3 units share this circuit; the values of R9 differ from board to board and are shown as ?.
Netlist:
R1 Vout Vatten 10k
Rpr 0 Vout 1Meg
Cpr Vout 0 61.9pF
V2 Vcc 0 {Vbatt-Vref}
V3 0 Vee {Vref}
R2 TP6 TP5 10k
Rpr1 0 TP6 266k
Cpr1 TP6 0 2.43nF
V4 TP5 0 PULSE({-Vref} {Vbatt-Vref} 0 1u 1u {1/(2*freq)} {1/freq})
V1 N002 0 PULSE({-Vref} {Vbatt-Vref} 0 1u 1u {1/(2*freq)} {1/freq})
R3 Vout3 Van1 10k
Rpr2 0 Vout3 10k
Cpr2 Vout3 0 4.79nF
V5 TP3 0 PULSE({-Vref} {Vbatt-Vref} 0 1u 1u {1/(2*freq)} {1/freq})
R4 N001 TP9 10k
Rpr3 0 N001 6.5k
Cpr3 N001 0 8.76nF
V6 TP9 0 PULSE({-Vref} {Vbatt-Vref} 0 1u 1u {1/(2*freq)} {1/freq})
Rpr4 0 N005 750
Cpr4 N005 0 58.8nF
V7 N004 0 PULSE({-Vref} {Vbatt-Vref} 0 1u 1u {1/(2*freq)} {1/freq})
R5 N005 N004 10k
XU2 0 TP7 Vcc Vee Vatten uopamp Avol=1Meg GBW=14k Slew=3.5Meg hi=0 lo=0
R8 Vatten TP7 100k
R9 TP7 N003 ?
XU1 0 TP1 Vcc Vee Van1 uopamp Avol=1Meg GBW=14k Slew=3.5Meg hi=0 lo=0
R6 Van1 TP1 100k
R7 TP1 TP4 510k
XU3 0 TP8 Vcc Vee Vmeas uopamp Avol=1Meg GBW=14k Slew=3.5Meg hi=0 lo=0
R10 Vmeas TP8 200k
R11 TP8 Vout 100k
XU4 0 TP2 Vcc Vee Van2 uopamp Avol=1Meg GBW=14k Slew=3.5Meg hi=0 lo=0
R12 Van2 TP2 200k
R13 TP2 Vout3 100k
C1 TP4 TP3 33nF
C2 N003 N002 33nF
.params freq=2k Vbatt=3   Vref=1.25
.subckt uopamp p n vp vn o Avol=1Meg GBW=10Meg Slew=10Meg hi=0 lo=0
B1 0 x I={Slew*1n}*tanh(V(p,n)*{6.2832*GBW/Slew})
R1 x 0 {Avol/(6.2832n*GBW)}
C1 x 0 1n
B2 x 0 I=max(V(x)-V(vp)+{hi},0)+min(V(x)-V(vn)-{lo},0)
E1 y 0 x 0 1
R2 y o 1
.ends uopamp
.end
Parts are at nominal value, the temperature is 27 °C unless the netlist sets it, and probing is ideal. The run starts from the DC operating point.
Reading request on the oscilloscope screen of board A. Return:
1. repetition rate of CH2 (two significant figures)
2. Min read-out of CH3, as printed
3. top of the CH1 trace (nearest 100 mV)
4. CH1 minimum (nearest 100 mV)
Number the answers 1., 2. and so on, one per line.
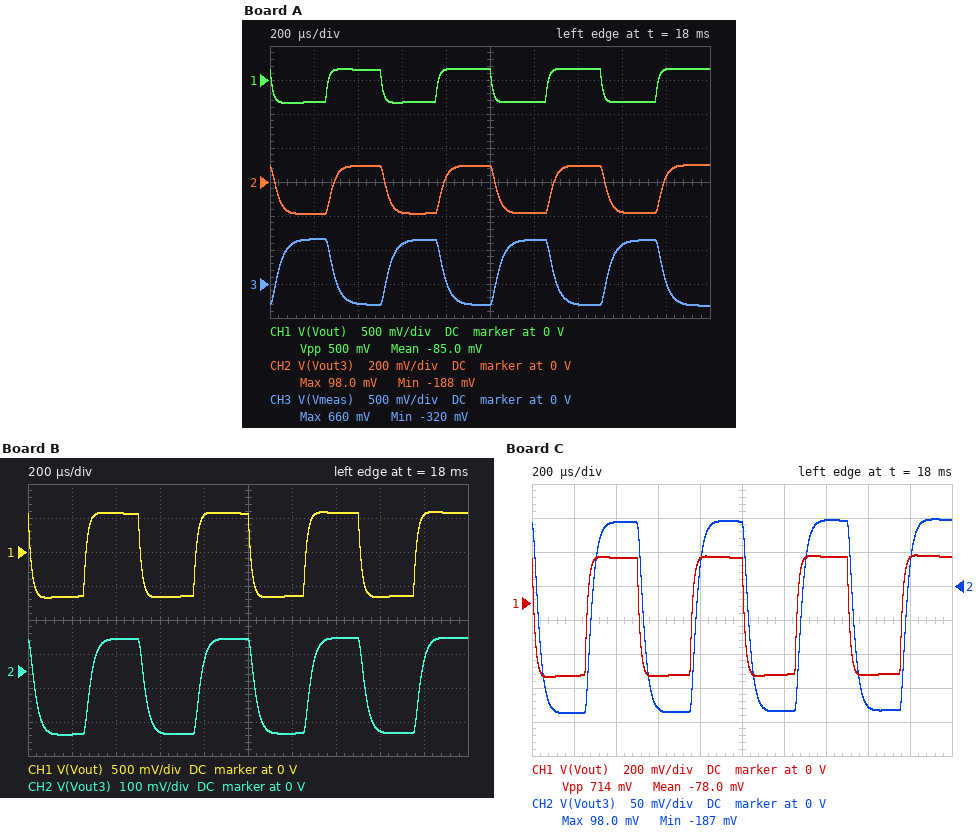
1. 2.0 kHz
2. -320 mV
3. 200 mV
4. -300 mV
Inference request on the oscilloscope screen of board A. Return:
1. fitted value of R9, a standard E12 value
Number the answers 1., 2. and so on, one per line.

1. 560 kΩ
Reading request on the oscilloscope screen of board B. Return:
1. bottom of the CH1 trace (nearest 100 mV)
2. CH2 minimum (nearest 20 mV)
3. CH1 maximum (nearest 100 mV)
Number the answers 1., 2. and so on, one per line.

1. -700 mV
2. -180 mV
3. 600 mV
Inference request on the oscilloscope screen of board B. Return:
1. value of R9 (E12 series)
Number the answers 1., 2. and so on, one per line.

1. 220 kΩ
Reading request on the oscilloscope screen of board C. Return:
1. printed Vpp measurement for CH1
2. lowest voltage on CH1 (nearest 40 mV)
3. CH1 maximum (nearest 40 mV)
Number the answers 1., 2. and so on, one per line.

1. 714 mV
2. -440 mV
3. 280 mV
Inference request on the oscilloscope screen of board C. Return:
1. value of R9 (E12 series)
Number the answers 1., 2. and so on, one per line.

1. 390 kΩ
